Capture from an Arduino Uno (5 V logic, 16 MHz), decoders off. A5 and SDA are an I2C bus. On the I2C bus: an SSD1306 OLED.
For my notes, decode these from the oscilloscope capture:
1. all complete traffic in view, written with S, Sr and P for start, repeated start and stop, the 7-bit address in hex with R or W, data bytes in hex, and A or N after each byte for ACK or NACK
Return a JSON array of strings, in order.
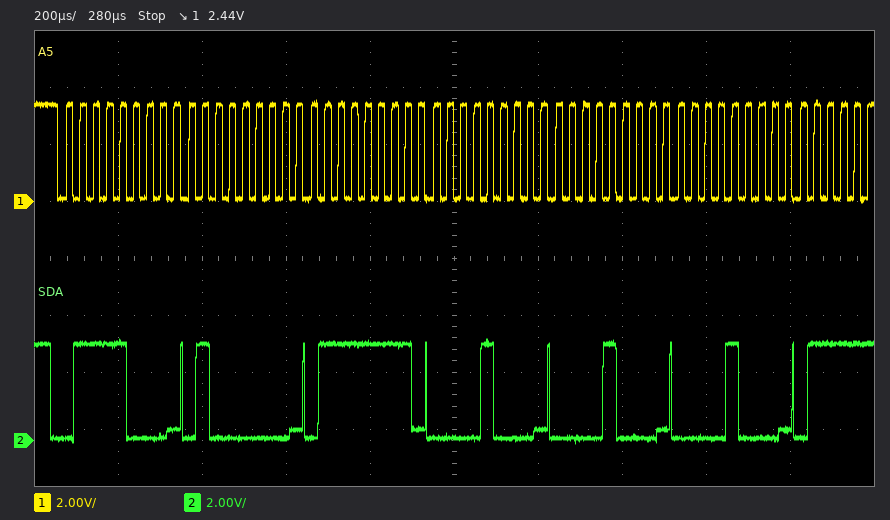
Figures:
["S 3CW A 40 A 7F A 08 A 08 A 08 A"]
